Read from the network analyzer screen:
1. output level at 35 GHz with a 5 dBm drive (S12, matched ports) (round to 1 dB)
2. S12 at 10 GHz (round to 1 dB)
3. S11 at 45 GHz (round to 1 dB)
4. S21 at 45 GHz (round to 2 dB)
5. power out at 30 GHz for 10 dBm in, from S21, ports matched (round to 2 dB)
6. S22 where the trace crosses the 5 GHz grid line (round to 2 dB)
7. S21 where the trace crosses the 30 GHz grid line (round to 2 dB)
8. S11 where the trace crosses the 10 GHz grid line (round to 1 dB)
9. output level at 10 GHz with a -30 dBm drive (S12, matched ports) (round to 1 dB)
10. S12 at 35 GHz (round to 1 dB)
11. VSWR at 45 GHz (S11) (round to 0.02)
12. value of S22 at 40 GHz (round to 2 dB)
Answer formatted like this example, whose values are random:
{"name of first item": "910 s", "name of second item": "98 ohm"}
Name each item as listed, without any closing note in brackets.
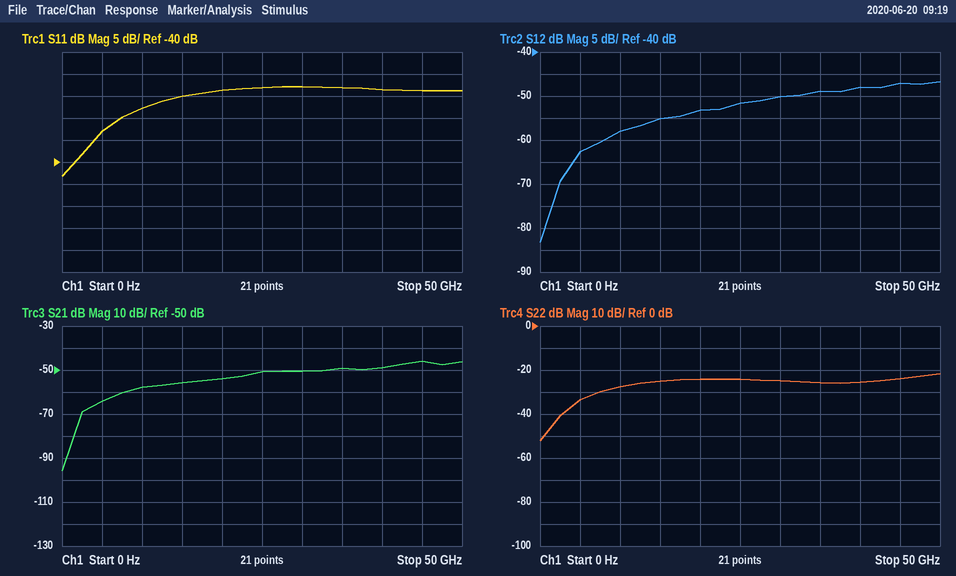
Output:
{"output level at 35 GHz with a 5 dBm drive (S12, matched ports)": "-44 dBm", "S12 at 10 GHz": "-58 dB", "S11 at 45 GHz": "-24 dB", "S21 at 45 GHz": "-46 dB", "power out at 30 GHz for 10 dBm in, from S21, ports matched": "-40 dBm", "S22 where the trace crosses the 5 GHz grid line": "-34 dB", "S21 where the trace crosses the 30 GHz grid line": "-50 dB", "S11 where the trace crosses the 10 GHz grid line": "-28 dB", "output level at 10 GHz with a -30 dBm drive (S12, matched ports)": "-88 dBm", "S12 at 35 GHz": "-49 dB", "VSWR at 45 GHz (S11)": "1.14", "value of S22 at 40 GHz": "-26 dB"}
